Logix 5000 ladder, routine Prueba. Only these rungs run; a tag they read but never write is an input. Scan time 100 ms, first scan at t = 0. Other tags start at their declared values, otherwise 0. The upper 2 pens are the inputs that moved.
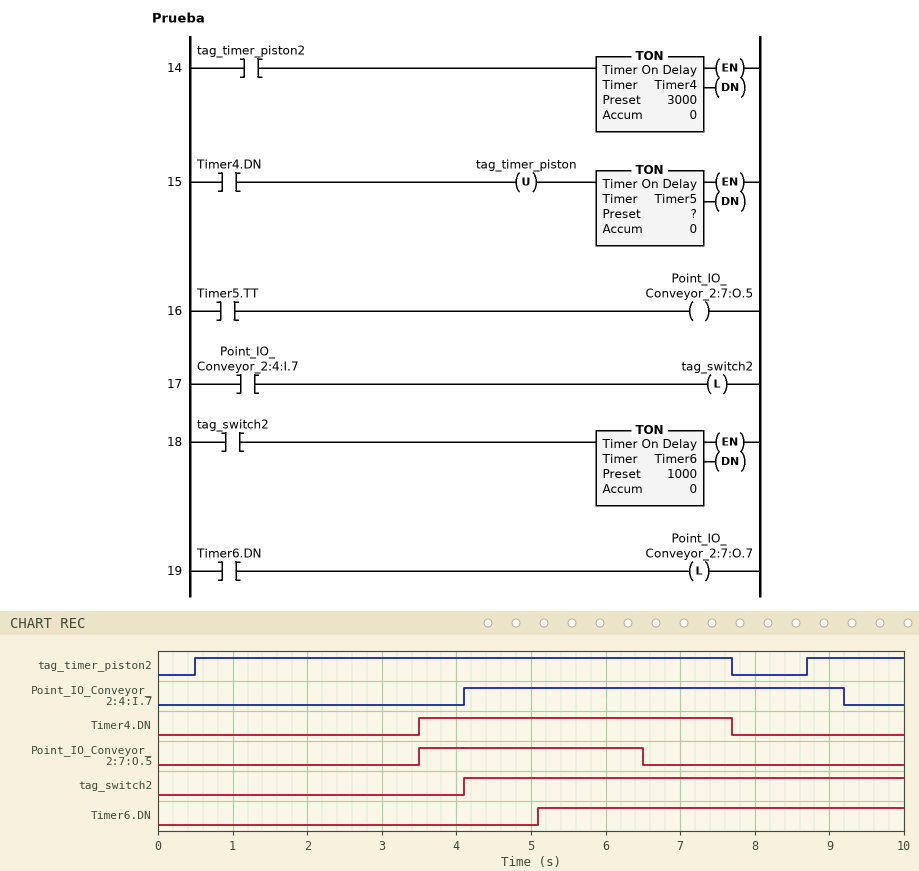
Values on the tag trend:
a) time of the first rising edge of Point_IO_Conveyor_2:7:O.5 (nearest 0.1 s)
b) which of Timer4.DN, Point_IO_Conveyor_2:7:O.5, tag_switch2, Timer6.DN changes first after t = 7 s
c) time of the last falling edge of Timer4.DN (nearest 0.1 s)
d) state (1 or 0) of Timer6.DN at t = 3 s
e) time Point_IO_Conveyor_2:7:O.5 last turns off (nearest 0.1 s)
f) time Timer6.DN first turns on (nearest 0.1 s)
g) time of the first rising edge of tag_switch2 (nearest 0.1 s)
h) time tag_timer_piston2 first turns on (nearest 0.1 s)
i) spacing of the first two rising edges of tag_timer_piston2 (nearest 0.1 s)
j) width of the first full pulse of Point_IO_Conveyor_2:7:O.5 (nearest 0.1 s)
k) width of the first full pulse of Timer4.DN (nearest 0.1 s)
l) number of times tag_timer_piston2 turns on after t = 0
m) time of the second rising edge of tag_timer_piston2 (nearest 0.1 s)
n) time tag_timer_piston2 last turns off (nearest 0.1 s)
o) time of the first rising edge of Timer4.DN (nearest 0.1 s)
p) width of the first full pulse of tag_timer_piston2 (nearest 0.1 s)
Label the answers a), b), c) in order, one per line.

a) 3.5 s
b) Timer4.DN
c) 7.7 s
d) 0
e) 6.5 s
f) 5.1 s
g) 4.1 s
h) 0.5 s
i) 8.2 s
j) 3.0 s
k) 4.2 s
l) 2
m) 8.7 s
n) 7.7 s
o) 3.5 s
p) 7.2 s
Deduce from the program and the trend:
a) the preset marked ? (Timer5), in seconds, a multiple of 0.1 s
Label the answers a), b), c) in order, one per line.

a) 3.0 s
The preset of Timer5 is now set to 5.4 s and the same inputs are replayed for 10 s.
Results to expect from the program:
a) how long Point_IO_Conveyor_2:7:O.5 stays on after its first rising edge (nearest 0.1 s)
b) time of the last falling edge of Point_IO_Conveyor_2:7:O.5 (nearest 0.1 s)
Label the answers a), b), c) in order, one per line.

a) 4.2 s
b) 7.7 s
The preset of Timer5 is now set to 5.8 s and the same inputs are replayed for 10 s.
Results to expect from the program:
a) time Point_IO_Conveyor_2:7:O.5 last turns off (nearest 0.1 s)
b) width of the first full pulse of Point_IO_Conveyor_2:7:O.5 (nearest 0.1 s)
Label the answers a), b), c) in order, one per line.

a) 7.7 s
b) 4.2 s
